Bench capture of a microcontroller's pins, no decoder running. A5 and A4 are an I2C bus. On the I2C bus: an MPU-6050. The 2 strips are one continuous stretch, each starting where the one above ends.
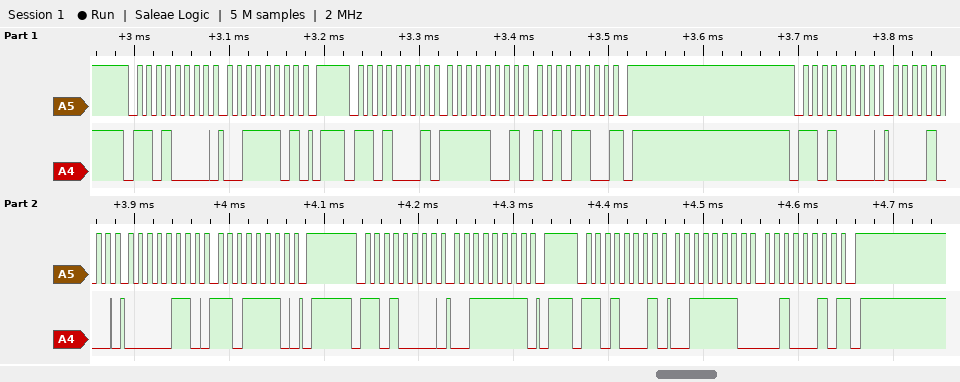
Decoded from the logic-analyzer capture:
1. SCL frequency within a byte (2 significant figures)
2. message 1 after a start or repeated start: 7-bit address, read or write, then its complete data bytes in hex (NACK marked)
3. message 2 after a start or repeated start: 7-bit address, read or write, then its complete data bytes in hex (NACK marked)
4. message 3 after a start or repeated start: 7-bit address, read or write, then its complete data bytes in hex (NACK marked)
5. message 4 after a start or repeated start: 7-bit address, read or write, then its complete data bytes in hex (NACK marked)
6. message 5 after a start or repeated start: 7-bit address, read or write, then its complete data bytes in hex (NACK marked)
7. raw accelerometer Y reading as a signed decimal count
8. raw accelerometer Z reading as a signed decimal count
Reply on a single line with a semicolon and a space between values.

100 kHz; 0x68 write: 3D; 0x68 read: F9 AC NACK; 0x68 write: 08 06 DE; 0x68 write: 3F; 0x68 read: 3E 22 NACK; -1620; 15906
